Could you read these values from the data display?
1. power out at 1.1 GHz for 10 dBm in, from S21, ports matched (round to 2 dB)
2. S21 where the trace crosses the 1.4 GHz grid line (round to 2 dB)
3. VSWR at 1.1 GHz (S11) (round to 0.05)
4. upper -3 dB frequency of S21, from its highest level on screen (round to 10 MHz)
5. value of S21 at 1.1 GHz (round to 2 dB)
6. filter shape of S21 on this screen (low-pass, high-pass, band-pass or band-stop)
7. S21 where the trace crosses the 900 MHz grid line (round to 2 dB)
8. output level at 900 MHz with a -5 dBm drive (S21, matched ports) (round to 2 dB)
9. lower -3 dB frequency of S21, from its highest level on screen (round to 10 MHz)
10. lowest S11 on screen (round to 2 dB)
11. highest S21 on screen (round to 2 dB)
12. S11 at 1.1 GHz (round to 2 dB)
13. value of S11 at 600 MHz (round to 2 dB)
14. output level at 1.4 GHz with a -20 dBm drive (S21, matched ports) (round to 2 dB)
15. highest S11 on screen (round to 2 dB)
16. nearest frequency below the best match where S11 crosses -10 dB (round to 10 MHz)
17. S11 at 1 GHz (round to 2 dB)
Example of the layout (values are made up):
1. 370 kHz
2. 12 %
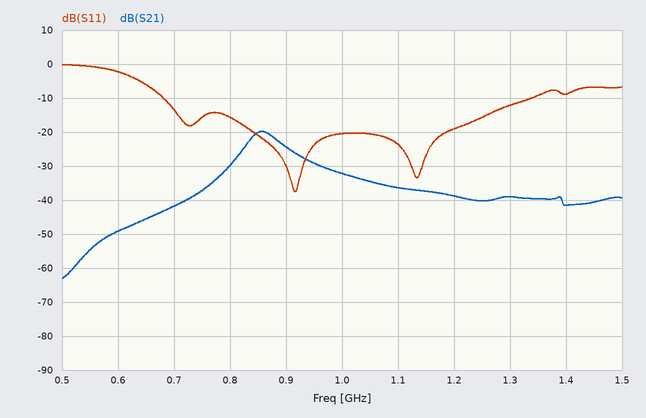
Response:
1. -26 dBm
2. -42 dB
3. 1.15
4. 890 MHz
5. -36 dB
6. band-pass
7. -24 dB
8. -30 dBm
9. 830 MHz
10. -38 dB
11. -20 dB
12. -24 dB
13. -2 dB
14. -62 dBm
15. 0 dB
16. 680 MHz
17. -20 dB
